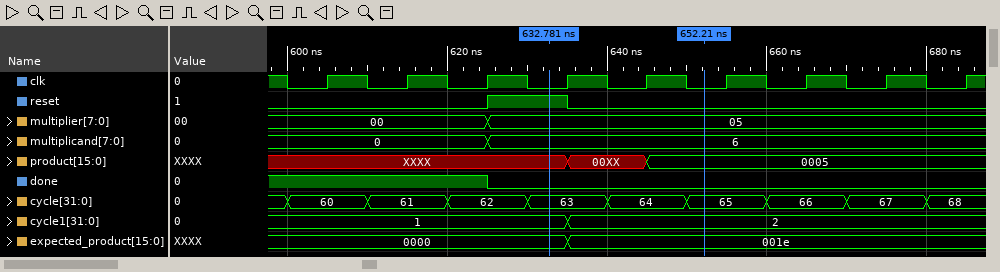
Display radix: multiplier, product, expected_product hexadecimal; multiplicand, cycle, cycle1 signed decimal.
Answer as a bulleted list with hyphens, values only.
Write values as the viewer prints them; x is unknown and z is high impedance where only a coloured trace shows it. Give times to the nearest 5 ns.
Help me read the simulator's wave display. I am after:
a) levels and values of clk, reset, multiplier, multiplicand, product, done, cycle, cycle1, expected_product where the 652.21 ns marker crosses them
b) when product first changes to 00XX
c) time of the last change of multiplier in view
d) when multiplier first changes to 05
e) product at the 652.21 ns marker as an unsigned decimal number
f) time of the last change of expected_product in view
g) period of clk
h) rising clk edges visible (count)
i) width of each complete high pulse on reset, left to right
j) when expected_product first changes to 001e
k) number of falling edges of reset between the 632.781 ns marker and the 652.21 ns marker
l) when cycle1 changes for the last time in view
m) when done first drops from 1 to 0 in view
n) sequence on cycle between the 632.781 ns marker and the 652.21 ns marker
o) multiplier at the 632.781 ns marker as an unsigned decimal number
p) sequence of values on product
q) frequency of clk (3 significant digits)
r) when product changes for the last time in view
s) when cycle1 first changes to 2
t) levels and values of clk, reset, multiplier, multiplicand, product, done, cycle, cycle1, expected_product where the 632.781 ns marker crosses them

- clk=0, reset=0, multiplier=05, multiplicand=6, product=0005, done=0, cycle=65, cycle1=2, expected_product=001e
- 635 ns
- 625 ns
- 625 ns
- 5
- 635 ns
- 10 ns
- 9
- 10 ns
- 635 ns
- 1
- 635 ns
- 625 ns
- 63, 64, 65
- 5
- XXXX, 00XX, 0005
- 100 MHz
- 645 ns
- 635 ns
- clk=0, reset=1, multiplier=05, multiplicand=6, product=XXXX, done=0, cycle=63, cycle1=1, expected_product=0000
